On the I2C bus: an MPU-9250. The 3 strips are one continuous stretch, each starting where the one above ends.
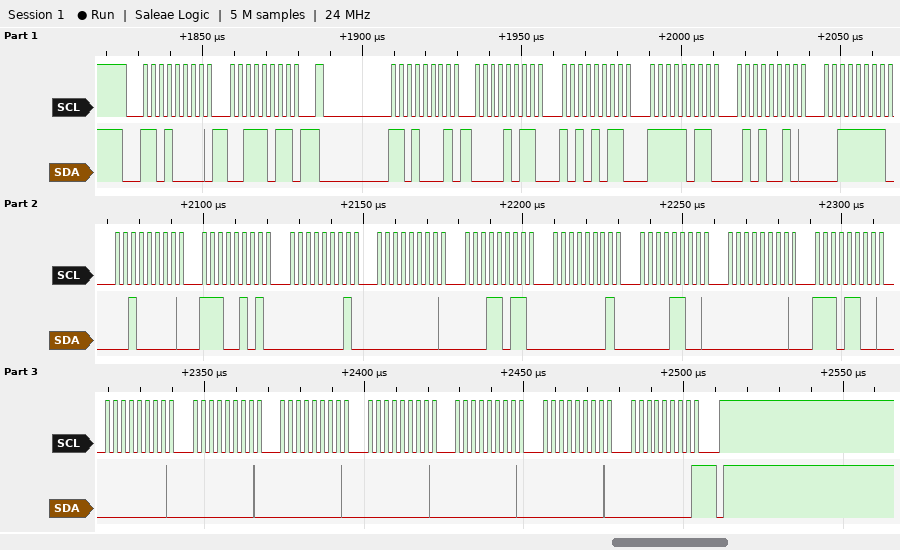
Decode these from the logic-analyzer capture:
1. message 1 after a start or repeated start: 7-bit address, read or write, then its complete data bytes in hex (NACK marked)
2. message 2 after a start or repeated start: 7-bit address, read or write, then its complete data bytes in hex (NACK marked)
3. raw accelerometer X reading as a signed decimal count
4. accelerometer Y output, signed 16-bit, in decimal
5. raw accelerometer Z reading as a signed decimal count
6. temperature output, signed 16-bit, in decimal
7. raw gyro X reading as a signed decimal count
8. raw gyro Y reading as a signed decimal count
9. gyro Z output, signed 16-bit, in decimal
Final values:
0x68 write: 3B
0x68 read: 0B AB FB 52 3F 20 E5 01 00 1B 01 0C 00 EC 00 00 00 00 00 00 00 NACK
2987
-1198
16160
-6911
27
268
236
